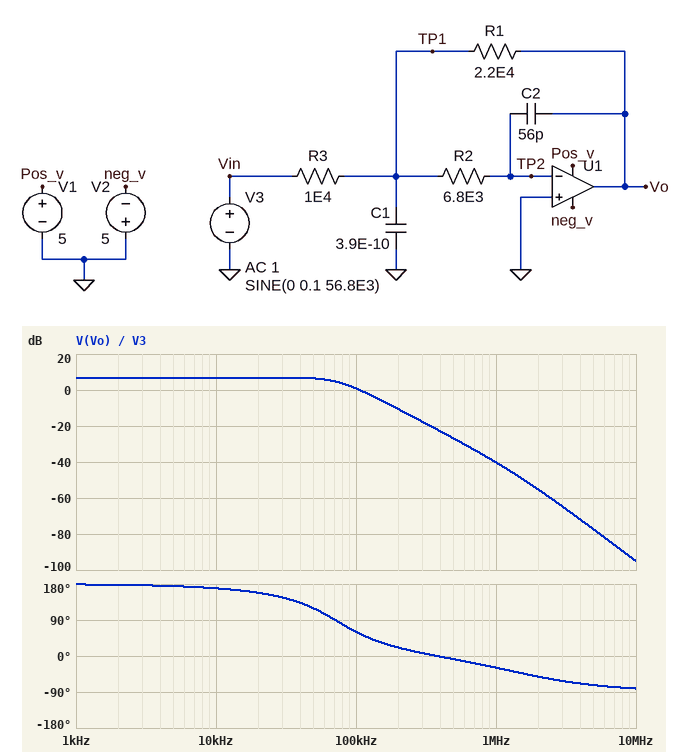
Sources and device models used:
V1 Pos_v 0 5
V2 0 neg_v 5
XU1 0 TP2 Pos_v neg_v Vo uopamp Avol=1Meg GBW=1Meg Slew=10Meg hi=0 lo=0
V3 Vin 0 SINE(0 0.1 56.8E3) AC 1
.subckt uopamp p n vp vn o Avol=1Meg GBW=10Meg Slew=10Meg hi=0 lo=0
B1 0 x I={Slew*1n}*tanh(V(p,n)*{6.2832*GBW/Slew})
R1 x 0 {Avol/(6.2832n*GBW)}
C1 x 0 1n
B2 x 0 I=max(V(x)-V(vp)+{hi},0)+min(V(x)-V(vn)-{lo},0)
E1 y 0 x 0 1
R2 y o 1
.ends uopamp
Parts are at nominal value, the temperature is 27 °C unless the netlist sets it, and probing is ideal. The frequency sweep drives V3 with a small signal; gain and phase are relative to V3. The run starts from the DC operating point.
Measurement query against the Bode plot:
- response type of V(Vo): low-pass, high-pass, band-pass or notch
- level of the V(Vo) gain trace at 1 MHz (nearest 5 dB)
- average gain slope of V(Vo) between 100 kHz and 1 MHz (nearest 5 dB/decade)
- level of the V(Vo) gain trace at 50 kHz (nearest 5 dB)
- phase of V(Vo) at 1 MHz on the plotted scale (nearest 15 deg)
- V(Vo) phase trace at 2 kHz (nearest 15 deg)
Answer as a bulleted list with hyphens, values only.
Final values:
- low-pass
- -40 dB
- -40 dB/decade
- 5 dB
- -30 deg
- 180 deg
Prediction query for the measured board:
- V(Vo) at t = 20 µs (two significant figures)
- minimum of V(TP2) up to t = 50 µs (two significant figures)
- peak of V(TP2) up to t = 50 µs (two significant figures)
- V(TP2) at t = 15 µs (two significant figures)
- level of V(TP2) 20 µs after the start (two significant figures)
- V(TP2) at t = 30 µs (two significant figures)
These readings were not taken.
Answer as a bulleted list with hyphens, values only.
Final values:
- 74 mV
- -11 mV
- 11 mV
- -6.3 mV
- 11 mV
- -11 mV
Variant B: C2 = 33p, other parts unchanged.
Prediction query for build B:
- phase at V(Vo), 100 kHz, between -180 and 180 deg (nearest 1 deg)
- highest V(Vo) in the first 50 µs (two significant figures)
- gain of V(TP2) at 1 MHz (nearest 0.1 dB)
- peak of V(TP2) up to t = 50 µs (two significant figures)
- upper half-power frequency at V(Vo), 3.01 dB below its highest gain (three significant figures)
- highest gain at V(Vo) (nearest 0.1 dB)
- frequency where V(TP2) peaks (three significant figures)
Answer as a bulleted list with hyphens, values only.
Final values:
- 71 deg
- 250 mV
- -36.8 dB
- 14 mV
- 101 kHz
- 8.0 dB
- 86.9 kHz
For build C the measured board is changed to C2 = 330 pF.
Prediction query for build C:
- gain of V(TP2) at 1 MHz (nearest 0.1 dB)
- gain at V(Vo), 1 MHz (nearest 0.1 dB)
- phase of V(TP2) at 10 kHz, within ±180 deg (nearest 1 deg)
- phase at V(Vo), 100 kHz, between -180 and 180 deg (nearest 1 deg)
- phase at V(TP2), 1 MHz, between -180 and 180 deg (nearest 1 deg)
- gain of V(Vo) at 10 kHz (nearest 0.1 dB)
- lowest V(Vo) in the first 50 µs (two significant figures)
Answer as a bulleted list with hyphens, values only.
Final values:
- -54.2 dB
- -54.1 dB
- 44 deg
- 47 deg
- -126 deg
- 4.5 dB
- -64 mV
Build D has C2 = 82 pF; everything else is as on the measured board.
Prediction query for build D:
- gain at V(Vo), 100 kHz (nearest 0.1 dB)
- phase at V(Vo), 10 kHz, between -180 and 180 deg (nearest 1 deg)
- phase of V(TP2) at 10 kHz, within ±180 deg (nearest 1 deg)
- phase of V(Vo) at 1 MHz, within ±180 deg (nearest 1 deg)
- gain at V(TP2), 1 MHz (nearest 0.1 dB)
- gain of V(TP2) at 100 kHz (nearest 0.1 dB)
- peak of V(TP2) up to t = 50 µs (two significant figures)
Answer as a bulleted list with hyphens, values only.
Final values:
- -2.4 dB
- 165 deg
- 75 deg
- -32 deg
- -43.0 dB
- -22.4 dB
- 8.7 mV
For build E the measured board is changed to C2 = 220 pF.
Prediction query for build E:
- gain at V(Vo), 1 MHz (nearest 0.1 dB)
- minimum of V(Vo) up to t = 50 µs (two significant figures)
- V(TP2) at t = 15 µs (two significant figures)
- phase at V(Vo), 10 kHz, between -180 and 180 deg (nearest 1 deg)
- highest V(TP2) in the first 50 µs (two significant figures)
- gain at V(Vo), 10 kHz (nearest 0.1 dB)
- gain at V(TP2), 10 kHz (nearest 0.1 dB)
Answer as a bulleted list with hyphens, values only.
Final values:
- -50.8 dB
- -88 mV
- -3.5 mV
- 146 deg
- 3.4 mV
- 5.8 dB
- -34.2 dB
